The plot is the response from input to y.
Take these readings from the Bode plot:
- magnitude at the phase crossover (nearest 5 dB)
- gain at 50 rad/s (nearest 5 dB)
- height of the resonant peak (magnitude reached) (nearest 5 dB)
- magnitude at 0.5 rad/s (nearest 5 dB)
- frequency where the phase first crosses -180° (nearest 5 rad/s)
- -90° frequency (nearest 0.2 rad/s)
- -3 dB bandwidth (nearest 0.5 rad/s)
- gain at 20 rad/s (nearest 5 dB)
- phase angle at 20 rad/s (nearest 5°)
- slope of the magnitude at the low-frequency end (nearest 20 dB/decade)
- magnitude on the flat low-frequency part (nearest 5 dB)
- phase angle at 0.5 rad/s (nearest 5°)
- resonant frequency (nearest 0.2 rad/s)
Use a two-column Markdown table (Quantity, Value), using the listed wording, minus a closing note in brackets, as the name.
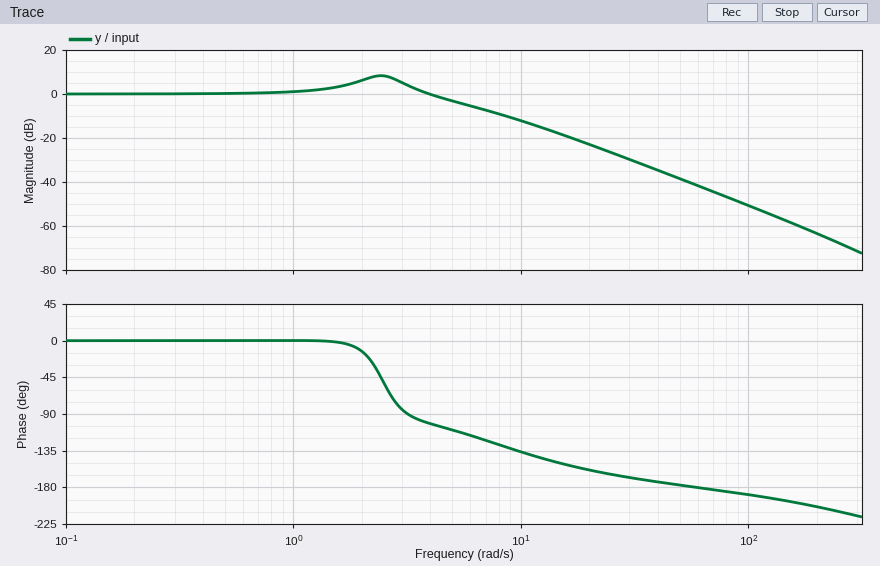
| Quantity | Value |
|---|---|
| magnitude at the phase crossover | -40 dB |
| gain at 50 rad/s | -40 dB |
| height of the resonant peak (magnitude reached) | 10 dB |
| magnitude at 0.5 rad/s | 0 dB |
| frequency where the phase first crosses -180° | 60 rad/s |
| -90° frequency | 3.2 rad/s |
| -3 dB bandwidth | 5.0 rad/s |
| gain at 20 rad/s | -25 dB |
| phase angle at 20 rad/s | -160° |
| slope of the magnitude at the low-frequency end | 0 dB/decade |
| magnitude on the flat low-frequency part | 0 dB |
| phase angle at 0.5 rad/s | 0° |
| resonant frequency | 2.4 rad/s |
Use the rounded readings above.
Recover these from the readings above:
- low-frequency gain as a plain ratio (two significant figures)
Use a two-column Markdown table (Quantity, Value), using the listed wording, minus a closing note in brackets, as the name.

| Quantity | Value |
|---|---|
| low-frequency gain as a plain ratio | 1.0 |
